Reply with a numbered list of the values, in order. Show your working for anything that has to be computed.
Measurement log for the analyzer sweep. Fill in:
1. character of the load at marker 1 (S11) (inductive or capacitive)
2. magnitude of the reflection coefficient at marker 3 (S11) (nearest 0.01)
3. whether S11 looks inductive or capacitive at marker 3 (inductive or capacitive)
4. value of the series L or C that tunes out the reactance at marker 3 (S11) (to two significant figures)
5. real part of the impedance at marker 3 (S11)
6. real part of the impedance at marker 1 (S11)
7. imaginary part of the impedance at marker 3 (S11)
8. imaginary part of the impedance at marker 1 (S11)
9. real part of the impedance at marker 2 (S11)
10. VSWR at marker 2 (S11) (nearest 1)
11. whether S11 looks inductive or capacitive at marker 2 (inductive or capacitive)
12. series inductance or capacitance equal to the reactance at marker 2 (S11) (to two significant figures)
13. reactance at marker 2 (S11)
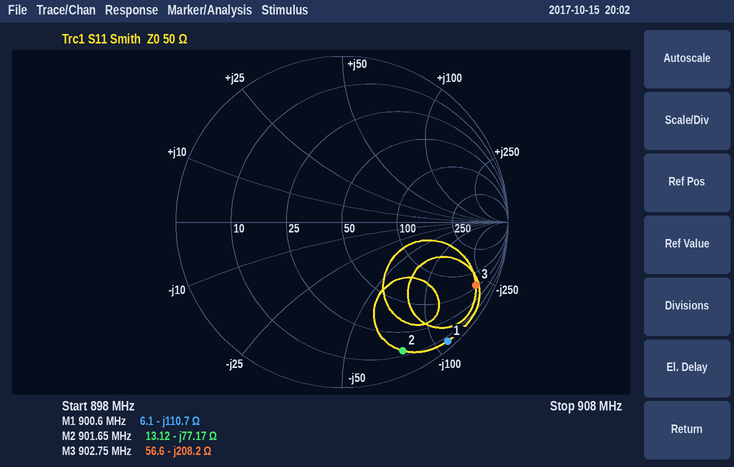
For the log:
1. capacitive
2. 0.89
3. capacitive
4. L = 208.2 Ω/(2π × 902.75 MHz) ≈ 37 nH
5. 56.6 Ω
6. 6.1 Ω
7. -208.2 Ω
8. -110.7 Ω
9. 13.12 Ω
10. 13
11. capacitive
12. C = 1/(2π × 901.65 MHz × 77.17 Ω) ≈ 2.3 pF
13. -77.17 Ω
